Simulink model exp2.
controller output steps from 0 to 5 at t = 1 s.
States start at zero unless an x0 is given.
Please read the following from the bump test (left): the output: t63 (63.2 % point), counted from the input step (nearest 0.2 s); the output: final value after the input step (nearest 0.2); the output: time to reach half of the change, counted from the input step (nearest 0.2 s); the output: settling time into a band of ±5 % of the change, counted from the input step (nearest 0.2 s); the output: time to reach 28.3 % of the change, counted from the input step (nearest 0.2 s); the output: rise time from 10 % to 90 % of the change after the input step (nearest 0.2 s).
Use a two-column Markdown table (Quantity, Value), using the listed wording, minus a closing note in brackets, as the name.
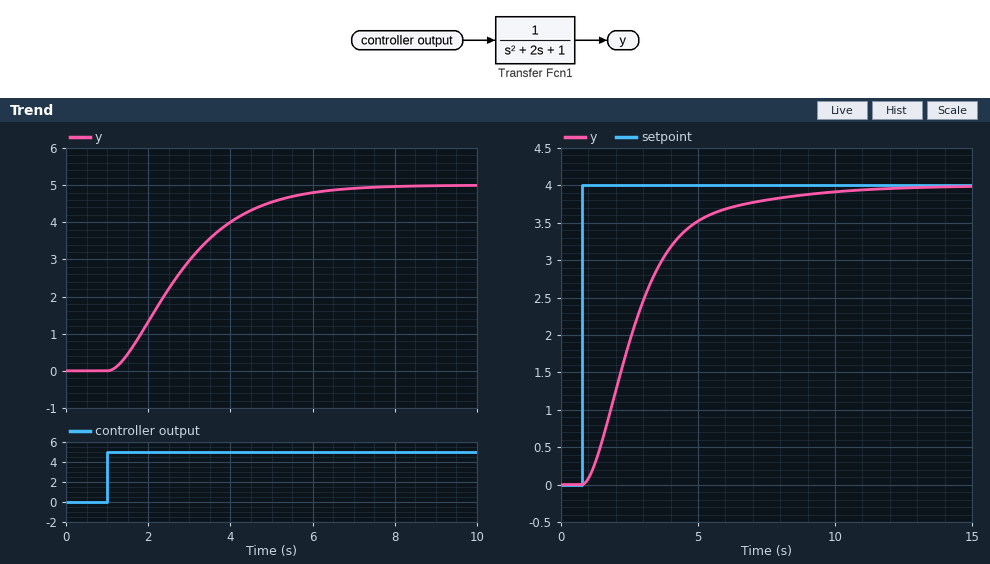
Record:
| Quantity | Value |
|---|---|
| the output: t63 (63.2 % point), counted from the input step | 2.2 s |
| the output: final value after the input step | 5.0 |
| the output: time to reach half of the change, counted from the input step | 1.6 s |
| the output: settling time into a band of ±5 % of the change, counted from the input step | 4.8 s |
| the output: time to reach 28.3 % of the change, counted from the input step | 1.0 s |
| the output: rise time from 10 % to 90 % of the change after the input step | 3.4 s |
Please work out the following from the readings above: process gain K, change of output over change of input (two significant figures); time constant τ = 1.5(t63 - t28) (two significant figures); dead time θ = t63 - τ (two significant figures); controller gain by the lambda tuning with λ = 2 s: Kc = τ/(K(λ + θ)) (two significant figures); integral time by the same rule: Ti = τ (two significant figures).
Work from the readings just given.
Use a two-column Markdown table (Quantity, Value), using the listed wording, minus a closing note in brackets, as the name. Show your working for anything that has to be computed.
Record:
| Quantity | Value |
|---|---|
| process gain K, change of output over change of input | (5 - 0) / 5 = 1.0 |
| time constant τ = 1.5(t63 - t28) | 1.5 × (2.2 - 1) = 1.8 s |
| dead time θ = t63 - τ | 2.2 - 1.8 = 0.40 s |
| controller gain by the lambda tuning with λ = 2 s: Kc = τ/(K(λ + θ)) | 1.8 / (1 × (2 + 0.4)) = 0.75 |
| integral time by the same rule: Ti = τ | 1.8 s |
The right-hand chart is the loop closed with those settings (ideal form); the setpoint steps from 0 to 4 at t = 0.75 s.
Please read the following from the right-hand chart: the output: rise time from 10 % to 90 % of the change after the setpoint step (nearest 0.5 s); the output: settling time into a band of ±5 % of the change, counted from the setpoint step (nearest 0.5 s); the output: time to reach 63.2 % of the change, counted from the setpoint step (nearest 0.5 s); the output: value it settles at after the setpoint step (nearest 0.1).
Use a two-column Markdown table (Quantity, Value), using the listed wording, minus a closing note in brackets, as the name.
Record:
| Quantity | Value |
|---|---|
| the output: rise time from 10 % to 90 % of the change after the setpoint step | 4.0 s |
| the output: settling time into a band of ±5 % of the change, counted from the setpoint step | 6.5 s |
| the output: time to reach 63.2 % of the change, counted from the setpoint step | 2.5 s |
| the output: value it settles at after the setpoint step | 4.0 |
